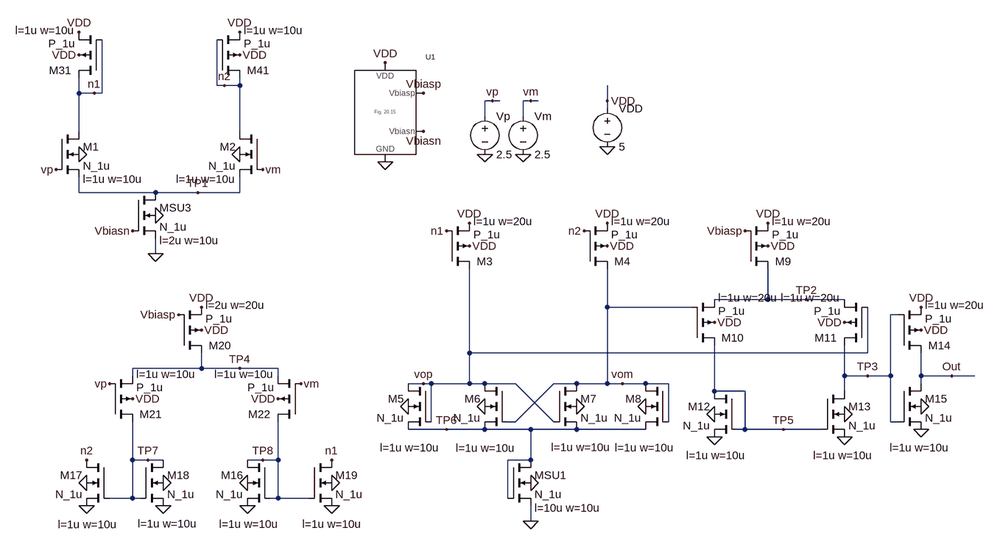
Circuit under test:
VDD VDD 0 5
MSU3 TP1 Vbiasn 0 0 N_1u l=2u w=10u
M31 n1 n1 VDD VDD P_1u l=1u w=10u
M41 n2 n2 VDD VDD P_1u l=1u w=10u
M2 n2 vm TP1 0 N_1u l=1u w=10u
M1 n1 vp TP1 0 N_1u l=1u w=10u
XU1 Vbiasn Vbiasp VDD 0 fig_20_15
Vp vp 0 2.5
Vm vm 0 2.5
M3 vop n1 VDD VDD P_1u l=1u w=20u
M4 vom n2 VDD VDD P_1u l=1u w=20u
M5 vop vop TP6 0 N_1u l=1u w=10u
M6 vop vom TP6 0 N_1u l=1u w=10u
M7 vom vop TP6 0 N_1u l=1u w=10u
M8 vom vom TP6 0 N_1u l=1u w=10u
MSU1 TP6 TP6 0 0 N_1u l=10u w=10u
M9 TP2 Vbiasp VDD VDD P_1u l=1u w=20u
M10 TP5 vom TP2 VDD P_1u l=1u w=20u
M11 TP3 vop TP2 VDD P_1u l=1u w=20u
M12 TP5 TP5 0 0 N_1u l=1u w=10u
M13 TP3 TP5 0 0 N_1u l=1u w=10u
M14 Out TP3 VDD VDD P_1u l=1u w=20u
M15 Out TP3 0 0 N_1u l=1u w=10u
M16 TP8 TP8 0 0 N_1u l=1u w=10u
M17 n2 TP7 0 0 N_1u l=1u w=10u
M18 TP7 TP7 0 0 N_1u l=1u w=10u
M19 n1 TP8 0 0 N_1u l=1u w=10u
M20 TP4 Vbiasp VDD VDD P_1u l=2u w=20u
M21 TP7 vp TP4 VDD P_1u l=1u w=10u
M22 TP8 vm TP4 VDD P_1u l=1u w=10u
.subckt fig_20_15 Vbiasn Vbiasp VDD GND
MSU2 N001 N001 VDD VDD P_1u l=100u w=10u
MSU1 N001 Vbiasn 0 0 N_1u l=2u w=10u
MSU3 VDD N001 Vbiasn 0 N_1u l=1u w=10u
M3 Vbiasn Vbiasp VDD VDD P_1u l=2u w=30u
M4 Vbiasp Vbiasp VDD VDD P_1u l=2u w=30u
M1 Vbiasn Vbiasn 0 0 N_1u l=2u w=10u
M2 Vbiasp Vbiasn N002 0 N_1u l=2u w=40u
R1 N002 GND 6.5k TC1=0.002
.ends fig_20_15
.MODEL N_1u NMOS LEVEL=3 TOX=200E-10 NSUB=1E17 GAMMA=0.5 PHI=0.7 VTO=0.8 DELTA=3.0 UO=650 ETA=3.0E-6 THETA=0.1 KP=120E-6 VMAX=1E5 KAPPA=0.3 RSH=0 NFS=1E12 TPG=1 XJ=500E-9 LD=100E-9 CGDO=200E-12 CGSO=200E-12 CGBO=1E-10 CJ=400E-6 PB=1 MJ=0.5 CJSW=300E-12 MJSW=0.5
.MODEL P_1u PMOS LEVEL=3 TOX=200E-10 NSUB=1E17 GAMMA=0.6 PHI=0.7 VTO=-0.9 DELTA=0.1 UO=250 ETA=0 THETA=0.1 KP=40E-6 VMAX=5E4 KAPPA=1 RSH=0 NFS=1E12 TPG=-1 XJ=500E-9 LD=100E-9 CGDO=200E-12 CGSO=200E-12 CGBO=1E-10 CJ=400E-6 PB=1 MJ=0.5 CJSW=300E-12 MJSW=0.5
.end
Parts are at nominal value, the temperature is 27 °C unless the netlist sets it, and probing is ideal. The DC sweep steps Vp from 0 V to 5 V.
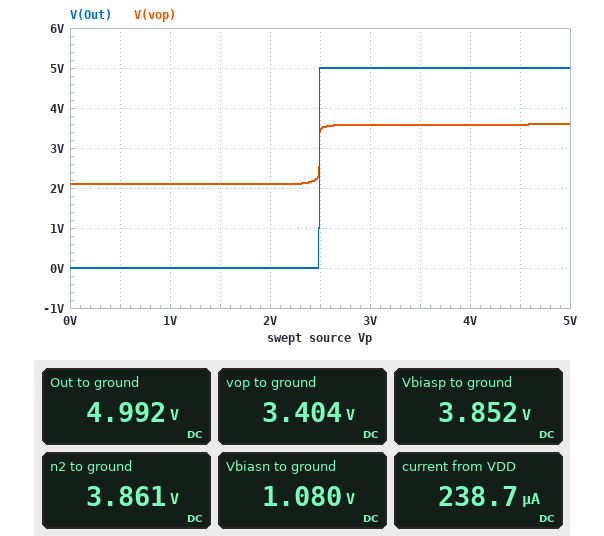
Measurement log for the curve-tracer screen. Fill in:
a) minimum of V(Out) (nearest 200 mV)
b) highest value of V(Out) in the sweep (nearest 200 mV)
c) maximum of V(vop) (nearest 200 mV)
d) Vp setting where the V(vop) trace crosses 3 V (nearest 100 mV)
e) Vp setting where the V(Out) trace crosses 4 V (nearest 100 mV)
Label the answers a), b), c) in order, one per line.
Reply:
a) 0 V
b) 5.0 V
c) 3.6 V
d) 2.5 V
e) 2.5 V
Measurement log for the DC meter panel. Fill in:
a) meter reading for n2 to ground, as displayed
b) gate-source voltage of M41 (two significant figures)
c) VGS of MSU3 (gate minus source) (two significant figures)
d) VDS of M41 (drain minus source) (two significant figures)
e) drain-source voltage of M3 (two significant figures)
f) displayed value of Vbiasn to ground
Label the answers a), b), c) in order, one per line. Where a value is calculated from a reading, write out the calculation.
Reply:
a) 3.861 V
b) 3.861 V - 5 V = -1.1 V
c) 1.08 V = 1.1 V
d) 3.861 V - 5 V = -1.1 V
e) 3.404 V - 5 V = -1.6 V
f) 1.080 V
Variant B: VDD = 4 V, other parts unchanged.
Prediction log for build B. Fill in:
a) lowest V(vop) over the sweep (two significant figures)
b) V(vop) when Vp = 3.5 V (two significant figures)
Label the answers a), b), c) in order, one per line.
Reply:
a) 2.0 V
b) 3.5 V
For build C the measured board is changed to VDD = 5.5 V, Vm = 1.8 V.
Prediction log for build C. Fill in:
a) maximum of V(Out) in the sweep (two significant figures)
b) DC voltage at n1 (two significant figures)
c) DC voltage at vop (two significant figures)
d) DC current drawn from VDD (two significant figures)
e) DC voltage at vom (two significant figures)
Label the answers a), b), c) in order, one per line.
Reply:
a) 5.5 V
b) 4.2 V
c) 3.6 V
d) 230 µA
e) 2.1 V
